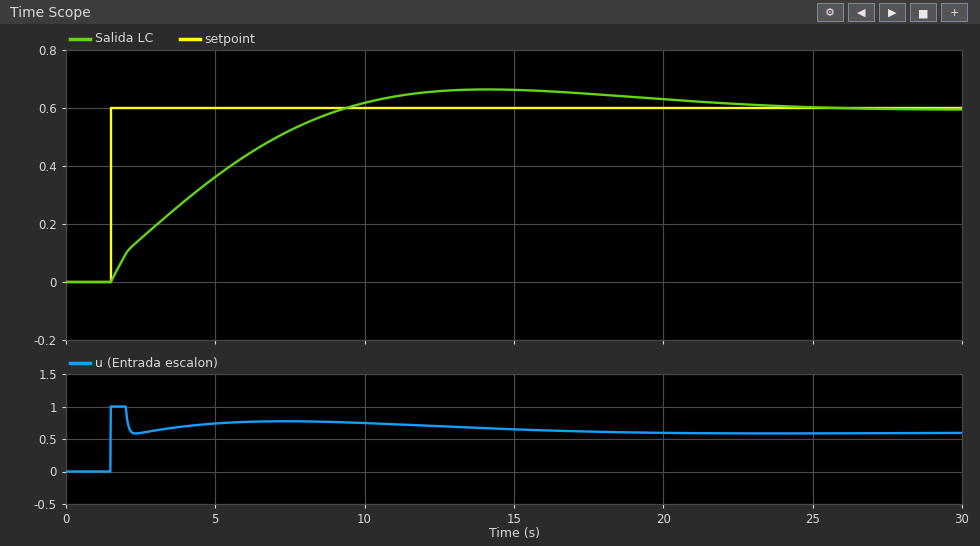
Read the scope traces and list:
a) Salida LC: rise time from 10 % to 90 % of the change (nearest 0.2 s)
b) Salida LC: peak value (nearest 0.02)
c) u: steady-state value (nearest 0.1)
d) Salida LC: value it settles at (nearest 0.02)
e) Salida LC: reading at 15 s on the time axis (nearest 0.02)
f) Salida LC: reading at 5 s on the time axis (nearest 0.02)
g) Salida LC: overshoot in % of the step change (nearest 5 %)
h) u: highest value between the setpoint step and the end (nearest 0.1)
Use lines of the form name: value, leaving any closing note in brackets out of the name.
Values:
Salida LC: rise time from 10 % to 90 % of the change: 6.0 s
Salida LC: peak value: 0.66
u: steady-state value: 0.6
Salida LC: value it settles at: 0.60
Salida LC: reading at 15 s on the time axis: 0.66
Salida LC: reading at 5 s on the time axis: 0.36
Salida LC: overshoot in % of the step change: 10 %
u: highest value between the setpoint step and the end: 1.0
